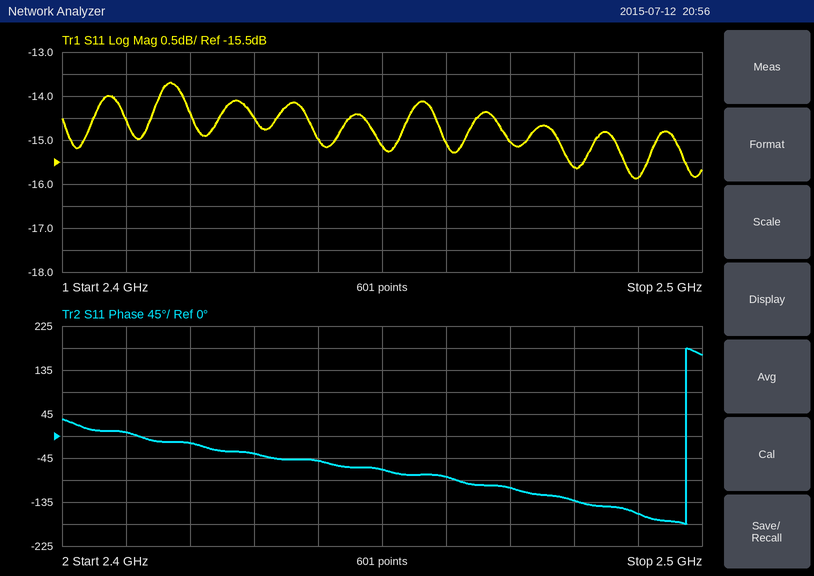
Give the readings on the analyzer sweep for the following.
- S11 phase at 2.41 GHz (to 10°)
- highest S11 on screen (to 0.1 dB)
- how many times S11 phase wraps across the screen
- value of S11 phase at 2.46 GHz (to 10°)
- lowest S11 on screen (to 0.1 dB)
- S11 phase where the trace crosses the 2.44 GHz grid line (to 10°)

10°
-13.7 dB
1
-80°
-15.9 dB
-50°
